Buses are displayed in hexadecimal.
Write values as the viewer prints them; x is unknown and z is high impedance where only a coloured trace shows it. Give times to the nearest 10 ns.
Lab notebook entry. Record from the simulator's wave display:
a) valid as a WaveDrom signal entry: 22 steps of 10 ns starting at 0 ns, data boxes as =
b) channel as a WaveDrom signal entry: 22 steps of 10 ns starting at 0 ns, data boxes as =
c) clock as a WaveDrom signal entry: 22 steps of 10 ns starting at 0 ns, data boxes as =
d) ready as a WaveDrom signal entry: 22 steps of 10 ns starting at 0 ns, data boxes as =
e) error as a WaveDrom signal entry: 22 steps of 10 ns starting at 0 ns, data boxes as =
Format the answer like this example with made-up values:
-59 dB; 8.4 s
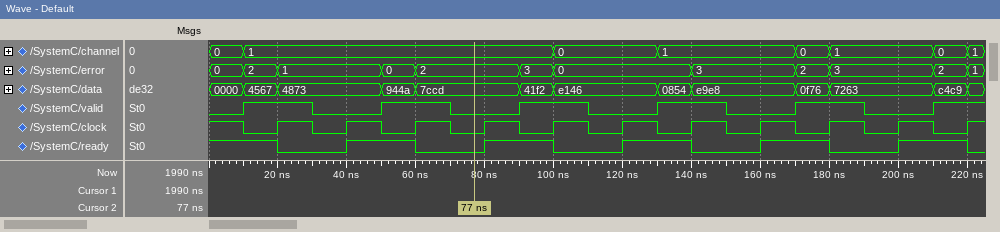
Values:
{name: 'valid', wave: '01.0.1.0.1.0.1.0.1.0.1'}; {name: 'channel', wave: '==........=..=...==..=', data: '0 1 0 1 0 1 0'}; {name: 'clock', wave: '1010101010101010101010'}; {name: 'ready', wave: '1.0.1.0.1.0.1.0.1.0.1.'}; {name: 'error', wave: '===..==..==...=..==..=', data: '0 2 1 0 2 3 0 3 2 3 2'}
